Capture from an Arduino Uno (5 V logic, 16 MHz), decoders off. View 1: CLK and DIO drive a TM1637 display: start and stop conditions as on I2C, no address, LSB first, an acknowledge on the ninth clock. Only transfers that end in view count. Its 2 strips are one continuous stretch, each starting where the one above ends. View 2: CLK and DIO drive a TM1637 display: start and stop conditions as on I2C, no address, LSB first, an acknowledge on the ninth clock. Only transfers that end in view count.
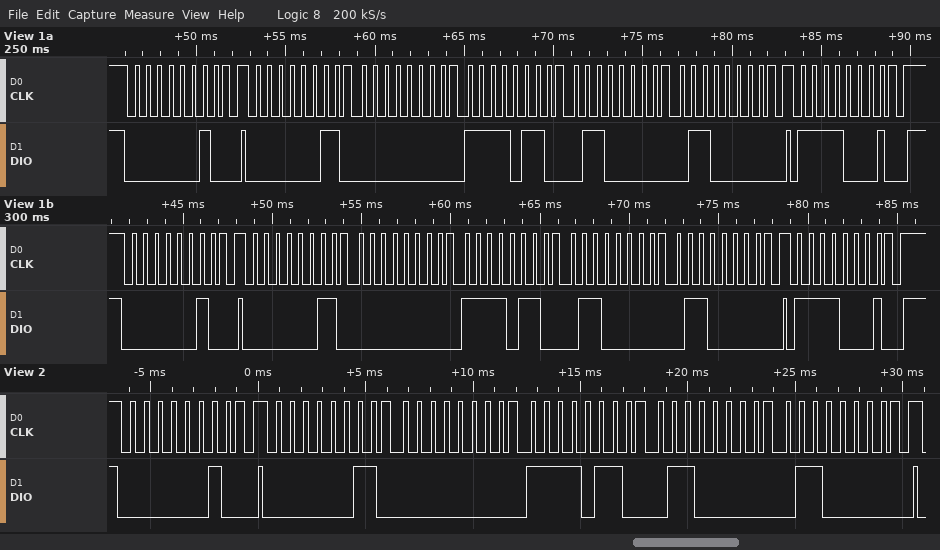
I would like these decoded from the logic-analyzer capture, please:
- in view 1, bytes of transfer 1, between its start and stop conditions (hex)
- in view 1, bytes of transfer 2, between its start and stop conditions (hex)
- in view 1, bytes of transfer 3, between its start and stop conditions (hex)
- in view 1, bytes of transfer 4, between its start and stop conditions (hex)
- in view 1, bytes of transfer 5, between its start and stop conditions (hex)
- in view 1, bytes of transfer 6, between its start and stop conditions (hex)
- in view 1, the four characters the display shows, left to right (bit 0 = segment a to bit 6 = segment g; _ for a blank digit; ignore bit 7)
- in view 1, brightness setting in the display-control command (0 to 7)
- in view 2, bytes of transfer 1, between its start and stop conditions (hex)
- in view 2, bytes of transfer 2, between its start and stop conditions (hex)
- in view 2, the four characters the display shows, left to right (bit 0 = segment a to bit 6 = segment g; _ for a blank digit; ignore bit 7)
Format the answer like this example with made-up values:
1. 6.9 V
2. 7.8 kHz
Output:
1. 40
2. C0 00 6F 06 06
3. 8F
4. 40
5. C0 00 6F 06 06
6. 8F
7. _911
8. 7
9. 40
10. C0 00 6F 06 06
11. _911
